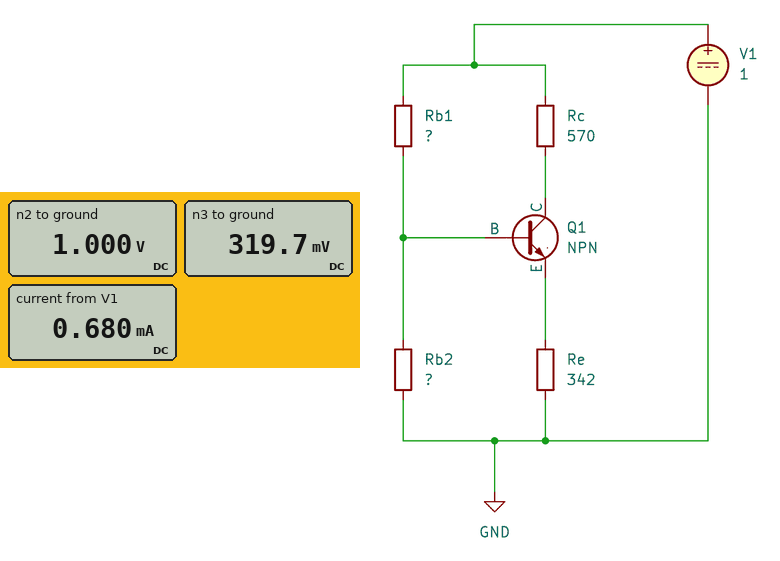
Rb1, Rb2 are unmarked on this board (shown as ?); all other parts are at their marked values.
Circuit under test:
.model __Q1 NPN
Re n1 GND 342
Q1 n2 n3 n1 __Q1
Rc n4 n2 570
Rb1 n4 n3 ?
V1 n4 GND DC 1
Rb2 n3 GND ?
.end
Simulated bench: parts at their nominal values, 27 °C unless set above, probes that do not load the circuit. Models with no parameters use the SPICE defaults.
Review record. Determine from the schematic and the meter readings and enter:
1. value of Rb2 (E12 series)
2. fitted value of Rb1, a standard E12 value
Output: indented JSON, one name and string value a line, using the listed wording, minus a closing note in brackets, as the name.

{
  "value of Rb2": "470 Ω",
  "fitted value of Rb1, a standard E12 value": "1 kΩ"
}
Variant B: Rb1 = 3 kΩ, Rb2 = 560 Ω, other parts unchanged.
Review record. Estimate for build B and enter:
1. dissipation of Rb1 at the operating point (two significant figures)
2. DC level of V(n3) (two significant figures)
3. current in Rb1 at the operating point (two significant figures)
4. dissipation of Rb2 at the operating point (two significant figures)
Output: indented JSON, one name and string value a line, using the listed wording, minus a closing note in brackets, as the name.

{
  "dissipation of Rb1 at the operating point": "240 µW",
  "DC level of V(n3)": "160 mV",
  "current in Rb1 at the operating point": "280 µA",
  "dissipation of Rb2 at the operating point": "44 µW"
}
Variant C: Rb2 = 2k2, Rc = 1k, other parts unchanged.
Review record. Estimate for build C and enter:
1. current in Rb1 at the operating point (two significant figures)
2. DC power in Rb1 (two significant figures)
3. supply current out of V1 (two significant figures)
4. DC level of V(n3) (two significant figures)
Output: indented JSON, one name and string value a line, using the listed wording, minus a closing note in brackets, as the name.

{
  "current in Rb1 at the operating point": "310 µA",
  "DC power in Rb1": "98 µW",
  "supply current out of V1": "340 µA",
  "DC level of V(n3)": "690 mV"
}
